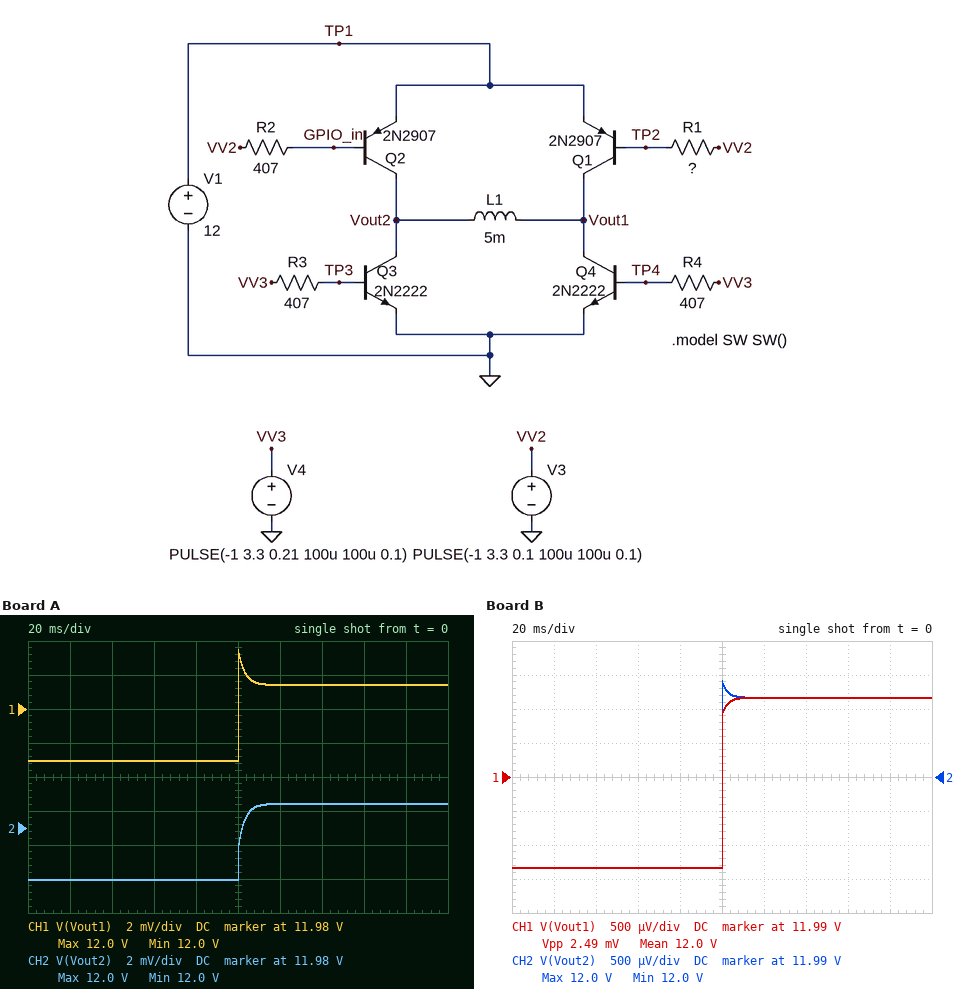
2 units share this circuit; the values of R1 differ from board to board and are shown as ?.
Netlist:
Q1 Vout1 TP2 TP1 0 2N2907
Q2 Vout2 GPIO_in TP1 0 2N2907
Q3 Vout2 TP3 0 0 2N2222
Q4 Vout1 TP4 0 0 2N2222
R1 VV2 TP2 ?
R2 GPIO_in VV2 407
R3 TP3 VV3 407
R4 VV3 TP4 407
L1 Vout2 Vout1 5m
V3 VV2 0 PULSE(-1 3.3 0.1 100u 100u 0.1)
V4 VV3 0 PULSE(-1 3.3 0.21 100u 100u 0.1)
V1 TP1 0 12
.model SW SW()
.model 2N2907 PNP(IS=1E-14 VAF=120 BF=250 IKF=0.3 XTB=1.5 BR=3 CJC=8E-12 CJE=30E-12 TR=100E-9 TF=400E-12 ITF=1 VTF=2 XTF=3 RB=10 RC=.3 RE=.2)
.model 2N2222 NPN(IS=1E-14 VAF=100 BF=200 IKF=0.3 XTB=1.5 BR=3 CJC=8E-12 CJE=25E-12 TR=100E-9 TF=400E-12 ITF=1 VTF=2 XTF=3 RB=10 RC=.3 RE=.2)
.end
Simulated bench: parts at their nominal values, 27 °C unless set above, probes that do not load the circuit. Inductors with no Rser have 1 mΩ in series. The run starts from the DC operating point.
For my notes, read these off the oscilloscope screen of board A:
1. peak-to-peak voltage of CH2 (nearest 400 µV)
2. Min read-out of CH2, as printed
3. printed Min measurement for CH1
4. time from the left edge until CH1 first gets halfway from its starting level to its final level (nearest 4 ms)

4.4 mV
12.0 V
12.0 V
100 ms
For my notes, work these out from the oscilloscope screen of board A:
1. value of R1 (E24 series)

160 Ω
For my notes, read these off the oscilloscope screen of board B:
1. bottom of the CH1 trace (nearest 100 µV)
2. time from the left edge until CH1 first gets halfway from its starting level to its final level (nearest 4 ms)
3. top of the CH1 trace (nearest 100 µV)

11.9852 V
100 ms
11.9877 V
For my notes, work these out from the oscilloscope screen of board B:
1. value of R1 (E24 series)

470 Ω
